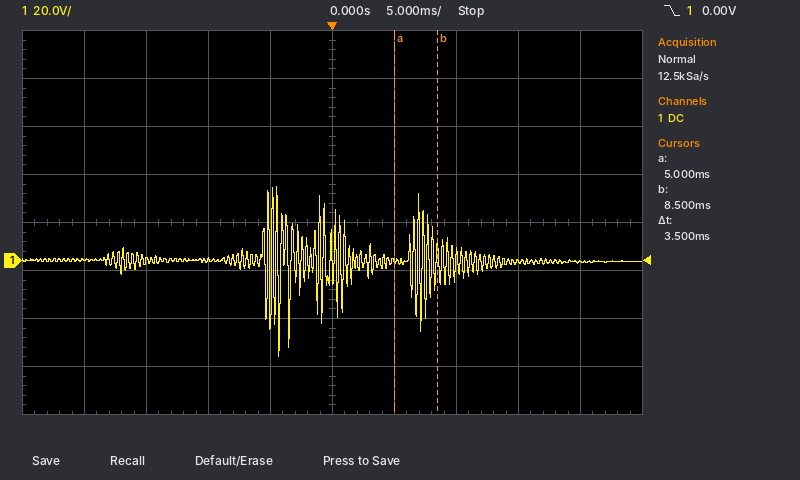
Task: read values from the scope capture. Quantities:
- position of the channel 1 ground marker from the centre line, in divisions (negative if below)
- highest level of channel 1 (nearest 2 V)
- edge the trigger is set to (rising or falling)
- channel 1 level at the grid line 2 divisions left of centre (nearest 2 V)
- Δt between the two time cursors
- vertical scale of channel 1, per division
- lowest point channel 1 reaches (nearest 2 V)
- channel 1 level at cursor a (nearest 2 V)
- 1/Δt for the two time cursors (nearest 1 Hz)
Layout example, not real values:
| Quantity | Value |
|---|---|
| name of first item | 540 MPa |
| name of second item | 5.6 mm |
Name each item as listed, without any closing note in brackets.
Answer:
| Quantity | Value |
|---|---|
| position of the channel 1 ground marker from the centre line, in divisions | -0.8 div |
| highest level of channel 1 | 32 V |
| edge the trigger is set to | falling |
| channel 1 level at the grid line 2 divisions left of centre | 0 V |
| Δt between the two time cursors | 3.5 ms |
| vertical scale of channel 1, per division | 20 V |
| lowest point channel 1 reaches | -40 V |
| channel 1 level at cursor a | 0 V |
| 1/Δt for the two time cursors | 286 Hz |
